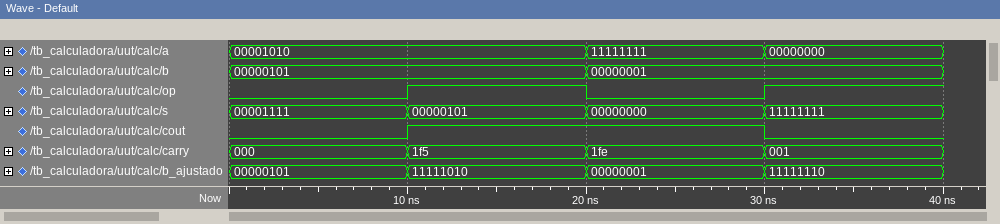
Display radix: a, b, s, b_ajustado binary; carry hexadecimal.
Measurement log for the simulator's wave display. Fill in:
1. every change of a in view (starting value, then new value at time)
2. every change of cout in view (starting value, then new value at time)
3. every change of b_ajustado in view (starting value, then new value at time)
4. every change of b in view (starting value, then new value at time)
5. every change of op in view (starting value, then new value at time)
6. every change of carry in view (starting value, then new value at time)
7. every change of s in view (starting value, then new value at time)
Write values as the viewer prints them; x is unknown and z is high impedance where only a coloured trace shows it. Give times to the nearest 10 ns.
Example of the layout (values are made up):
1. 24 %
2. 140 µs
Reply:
1. 00001010, 11111111 at 20 ns, 00000000 at 30 ns
2. 0, 1 at 10 ns, 0 at 30 ns
3. 00000101, 11111010 at 10 ns, 00000001 at 20 ns, 11111110 at 30 ns
4. 00000101, 00000001 at 20 ns
5. 0, 1 at 10 ns, 0 at 20 ns, 1 at 30 ns
6. 000, 1f5 at 10 ns, 1fe at 20 ns, 001 at 30 ns
7. 00001111, 00000101 at 10 ns, 00000000 at 20 ns, 11111111 at 30 ns
